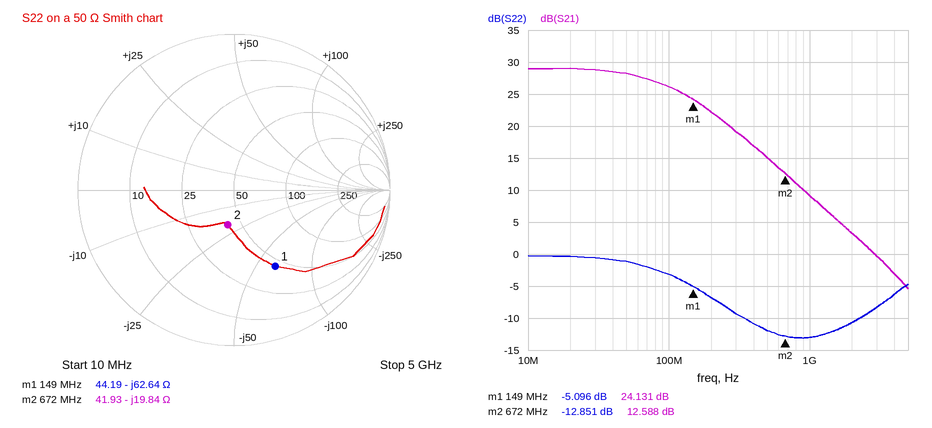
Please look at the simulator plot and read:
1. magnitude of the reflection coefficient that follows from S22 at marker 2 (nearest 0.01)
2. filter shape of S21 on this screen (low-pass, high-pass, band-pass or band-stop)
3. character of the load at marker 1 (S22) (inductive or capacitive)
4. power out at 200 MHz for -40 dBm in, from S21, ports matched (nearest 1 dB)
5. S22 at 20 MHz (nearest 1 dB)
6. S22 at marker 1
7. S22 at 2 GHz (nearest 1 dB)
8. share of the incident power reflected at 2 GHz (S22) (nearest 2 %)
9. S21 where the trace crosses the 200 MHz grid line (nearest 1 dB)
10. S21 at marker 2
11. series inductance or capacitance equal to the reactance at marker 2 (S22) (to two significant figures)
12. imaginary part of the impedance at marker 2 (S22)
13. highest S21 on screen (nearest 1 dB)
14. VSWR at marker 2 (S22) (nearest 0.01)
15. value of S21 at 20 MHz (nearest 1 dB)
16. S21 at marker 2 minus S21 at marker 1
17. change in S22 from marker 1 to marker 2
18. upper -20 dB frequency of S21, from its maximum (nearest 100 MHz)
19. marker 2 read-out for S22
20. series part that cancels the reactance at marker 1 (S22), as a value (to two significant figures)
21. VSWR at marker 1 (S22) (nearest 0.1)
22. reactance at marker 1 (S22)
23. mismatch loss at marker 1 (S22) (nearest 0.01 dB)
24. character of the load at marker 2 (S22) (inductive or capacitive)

0.23
low-pass
capacitive
-18 dBm
0 dB
-5.096 dB
-11 dB
8 %
22 dB
12.588 dB
12 pF
-19.84 Ω
29 dB
1.59
29 dB
-11.543 dB
-7.755 dB
1.0 GHz
-12.851 dB
67 nH
3.5
-62.64 Ω
1.61 dB
capacitive
